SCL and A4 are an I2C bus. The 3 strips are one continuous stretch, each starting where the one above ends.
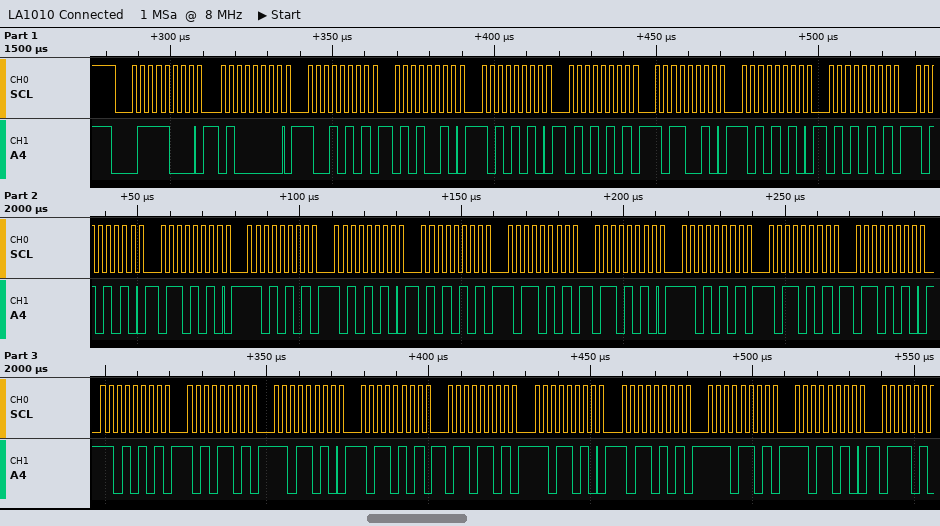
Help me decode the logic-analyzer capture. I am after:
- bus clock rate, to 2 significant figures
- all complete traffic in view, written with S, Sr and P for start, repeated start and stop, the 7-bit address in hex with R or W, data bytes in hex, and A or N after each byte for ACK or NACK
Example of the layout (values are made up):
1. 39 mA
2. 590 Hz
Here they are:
1. 400 kHz
2. S 3CW A 40 A 95 A 52 A AA A 55 A B2 A AA A 55 A AA A 6A A D5 A AA A 55 A B5 A 6A A D5 A B5 A 6A A D5 A AD A DA A B5 A 6D A DA A B5 A ED A DA A
